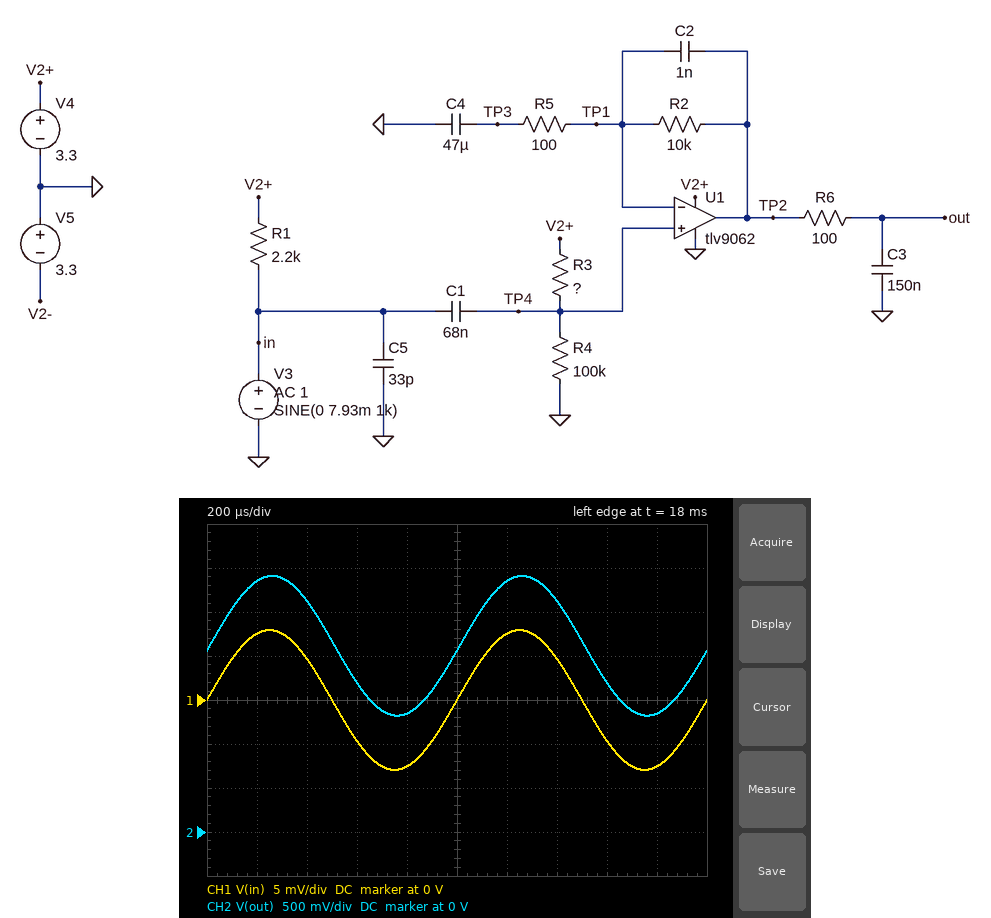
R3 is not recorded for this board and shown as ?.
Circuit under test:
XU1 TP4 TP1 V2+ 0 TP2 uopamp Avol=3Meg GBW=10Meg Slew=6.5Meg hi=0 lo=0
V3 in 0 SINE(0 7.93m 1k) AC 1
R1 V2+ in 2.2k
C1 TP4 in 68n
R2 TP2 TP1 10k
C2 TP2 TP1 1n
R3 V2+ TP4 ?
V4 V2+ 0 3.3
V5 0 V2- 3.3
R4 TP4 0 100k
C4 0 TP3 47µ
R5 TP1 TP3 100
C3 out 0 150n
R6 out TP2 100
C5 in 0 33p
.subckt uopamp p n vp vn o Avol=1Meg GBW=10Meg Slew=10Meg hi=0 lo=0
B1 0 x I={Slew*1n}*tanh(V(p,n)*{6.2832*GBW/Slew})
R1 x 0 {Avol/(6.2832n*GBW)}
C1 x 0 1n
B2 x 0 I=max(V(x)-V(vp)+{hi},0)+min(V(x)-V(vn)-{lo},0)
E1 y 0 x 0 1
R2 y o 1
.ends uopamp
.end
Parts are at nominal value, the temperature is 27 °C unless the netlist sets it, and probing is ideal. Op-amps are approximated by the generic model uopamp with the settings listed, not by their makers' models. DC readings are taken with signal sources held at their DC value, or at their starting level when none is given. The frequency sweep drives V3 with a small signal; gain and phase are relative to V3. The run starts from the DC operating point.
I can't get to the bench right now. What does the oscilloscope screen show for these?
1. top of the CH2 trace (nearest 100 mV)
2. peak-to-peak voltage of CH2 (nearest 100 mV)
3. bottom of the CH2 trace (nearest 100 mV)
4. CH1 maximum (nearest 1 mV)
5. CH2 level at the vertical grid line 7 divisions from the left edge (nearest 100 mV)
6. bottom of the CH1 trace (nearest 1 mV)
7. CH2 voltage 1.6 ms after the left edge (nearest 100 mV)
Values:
2.9 V
1.6 V
1.3 V
8 mV
2.6 V
-8 mV
1.7 V
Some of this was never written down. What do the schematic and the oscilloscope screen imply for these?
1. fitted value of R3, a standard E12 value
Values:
56 kΩ
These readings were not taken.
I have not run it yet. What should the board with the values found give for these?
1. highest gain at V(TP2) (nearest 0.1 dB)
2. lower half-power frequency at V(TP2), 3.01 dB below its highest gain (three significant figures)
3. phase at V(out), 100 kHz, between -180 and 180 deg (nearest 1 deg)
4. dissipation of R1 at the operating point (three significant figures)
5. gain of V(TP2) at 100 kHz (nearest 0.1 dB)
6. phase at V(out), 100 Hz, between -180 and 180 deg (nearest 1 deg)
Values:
40.0 dB
77.9 Hz
-163 deg
4.95 mW
22.8 dB
51 deg
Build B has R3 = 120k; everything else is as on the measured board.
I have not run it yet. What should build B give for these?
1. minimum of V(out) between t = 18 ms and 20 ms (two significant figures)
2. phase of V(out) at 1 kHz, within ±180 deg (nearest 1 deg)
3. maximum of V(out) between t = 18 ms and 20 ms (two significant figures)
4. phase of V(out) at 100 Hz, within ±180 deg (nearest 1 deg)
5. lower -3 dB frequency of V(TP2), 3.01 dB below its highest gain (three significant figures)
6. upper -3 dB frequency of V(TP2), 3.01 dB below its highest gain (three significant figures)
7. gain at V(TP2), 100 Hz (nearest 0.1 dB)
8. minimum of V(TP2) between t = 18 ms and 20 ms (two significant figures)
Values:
710 mV
-5 deg
2.3 V
41 deg
59.4 Hz
13.8 kHz
38.9 dB
700 mV
